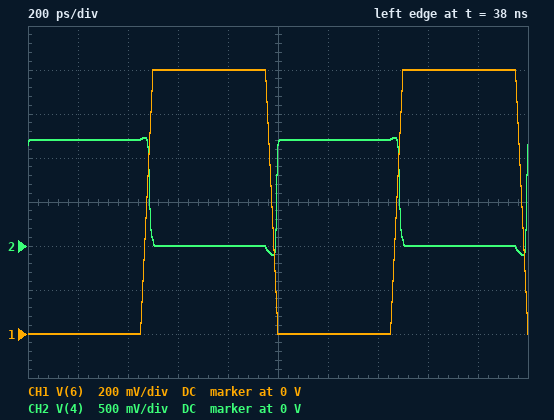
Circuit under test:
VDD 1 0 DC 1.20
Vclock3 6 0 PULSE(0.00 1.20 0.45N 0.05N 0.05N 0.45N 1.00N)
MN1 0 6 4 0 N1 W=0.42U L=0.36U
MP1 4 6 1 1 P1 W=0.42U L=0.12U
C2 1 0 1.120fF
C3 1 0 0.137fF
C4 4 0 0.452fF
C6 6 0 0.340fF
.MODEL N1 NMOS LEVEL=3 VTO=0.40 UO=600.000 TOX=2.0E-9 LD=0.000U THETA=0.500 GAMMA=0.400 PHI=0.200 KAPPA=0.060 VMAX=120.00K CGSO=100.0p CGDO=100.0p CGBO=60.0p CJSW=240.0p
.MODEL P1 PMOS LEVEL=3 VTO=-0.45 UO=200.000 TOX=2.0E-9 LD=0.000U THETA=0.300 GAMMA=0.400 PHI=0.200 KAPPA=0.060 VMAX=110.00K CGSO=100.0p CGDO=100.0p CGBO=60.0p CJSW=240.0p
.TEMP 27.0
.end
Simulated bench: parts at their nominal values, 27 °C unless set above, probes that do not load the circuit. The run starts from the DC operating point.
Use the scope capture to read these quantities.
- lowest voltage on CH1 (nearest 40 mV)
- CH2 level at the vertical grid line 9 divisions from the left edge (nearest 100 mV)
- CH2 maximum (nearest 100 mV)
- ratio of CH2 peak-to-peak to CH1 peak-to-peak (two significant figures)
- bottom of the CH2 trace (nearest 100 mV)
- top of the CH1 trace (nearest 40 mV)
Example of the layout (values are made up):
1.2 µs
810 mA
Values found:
0 V
0 V
1.2 V
1.1
-100 mV
1.20 V
